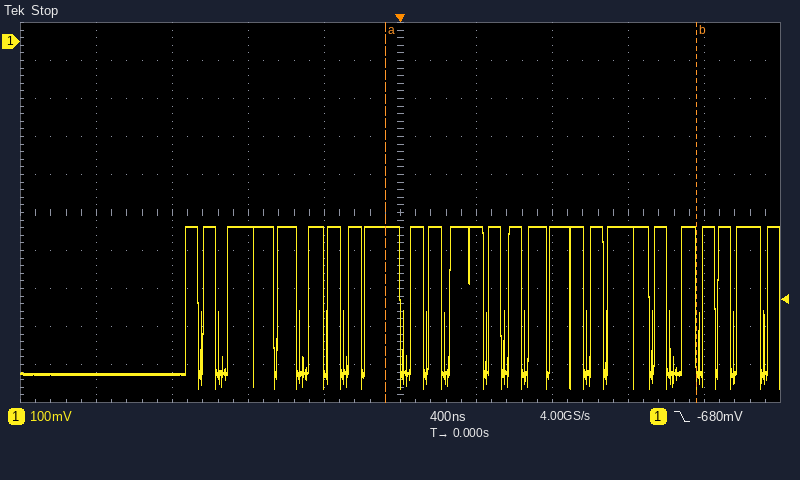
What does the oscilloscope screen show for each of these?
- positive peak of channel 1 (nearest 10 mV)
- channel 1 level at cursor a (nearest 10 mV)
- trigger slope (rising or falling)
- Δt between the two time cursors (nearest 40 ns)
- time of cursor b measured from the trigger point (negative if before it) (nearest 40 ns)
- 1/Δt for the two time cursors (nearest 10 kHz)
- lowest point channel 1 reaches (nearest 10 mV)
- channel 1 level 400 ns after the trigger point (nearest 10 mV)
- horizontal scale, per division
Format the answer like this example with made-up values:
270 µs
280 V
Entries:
-490 mV
-490 mV
falling
1.64 µs
+1.56 µs
610 kHz
-910 mV
-490 mV
400 ns
